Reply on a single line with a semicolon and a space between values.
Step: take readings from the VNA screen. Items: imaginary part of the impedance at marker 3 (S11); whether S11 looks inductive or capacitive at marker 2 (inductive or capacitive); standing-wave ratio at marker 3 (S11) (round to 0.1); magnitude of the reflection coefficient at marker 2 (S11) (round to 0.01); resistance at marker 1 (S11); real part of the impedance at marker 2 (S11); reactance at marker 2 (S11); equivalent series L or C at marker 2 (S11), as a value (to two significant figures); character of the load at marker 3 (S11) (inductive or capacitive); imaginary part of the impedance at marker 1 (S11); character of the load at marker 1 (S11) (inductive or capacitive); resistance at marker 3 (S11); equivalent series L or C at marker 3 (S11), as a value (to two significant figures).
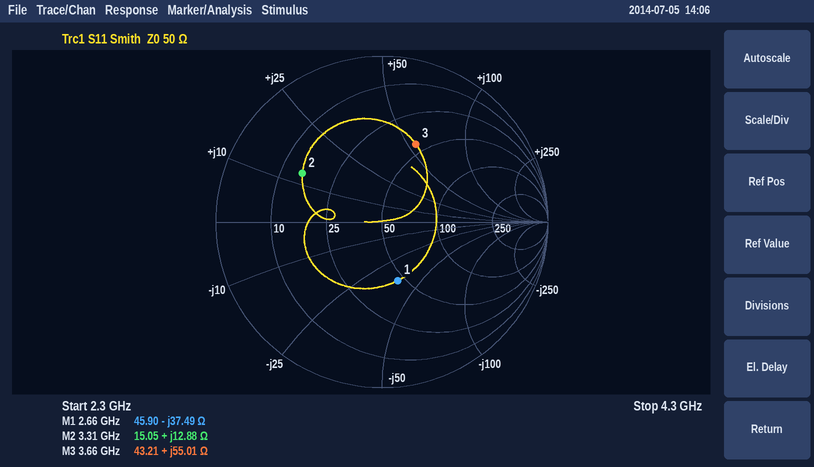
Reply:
+55.01 Ω; inductive; 3.1; 0.56; 45.90 Ω; 15.05 Ω; +12.88 Ω; 620 pH; inductive; -37.49 Ω; capacitive; 43.21 Ω; 2.4 nH
